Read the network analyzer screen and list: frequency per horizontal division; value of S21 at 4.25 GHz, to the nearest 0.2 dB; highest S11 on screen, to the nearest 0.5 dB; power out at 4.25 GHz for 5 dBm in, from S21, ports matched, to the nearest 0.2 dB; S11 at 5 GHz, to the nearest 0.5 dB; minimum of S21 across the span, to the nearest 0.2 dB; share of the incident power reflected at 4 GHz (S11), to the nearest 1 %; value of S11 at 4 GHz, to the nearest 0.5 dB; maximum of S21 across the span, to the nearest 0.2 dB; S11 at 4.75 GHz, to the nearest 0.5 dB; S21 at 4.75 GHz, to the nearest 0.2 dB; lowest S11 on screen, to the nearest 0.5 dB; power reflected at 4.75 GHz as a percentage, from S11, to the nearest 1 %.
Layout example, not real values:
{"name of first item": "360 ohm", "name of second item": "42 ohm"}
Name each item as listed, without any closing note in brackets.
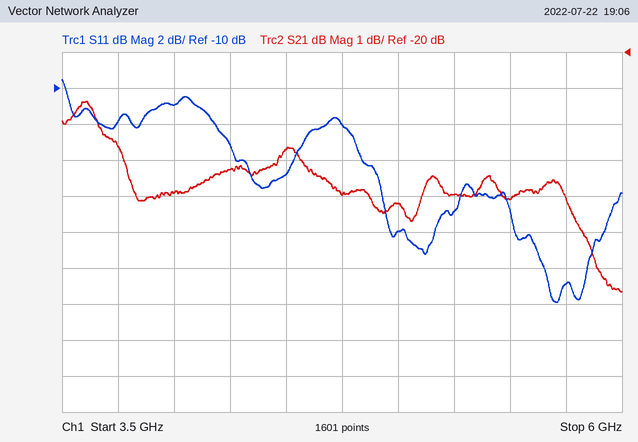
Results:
{"frequency per horizontal division": "250 MHz", "value of S21 at 4.25 GHz, to the nearest 0.2 dB": "-23.2 dB", "highest S11 on screen, to the nearest 0.5 dB": "-9.5 dB", "power out at 4.25 GHz for 5 dBm in, from S21, ports matched, to the nearest 0.2 dB": "-18.2 dBm", "S11 at 5 GHz, to the nearest 0.5 dB": "-18.0 dB", "minimum of S21 across the span, to the nearest 0.2 dB": "-26.6 dB", "share of the incident power reflected at 4 GHz (S11), to the nearest 1 %": "8 %", "value of S11 at 4 GHz, to the nearest 0.5 dB": "-11.0 dB", "maximum of S21 across the span, to the nearest 0.2 dB": "-21.4 dB", "S11 at 4.75 GHz, to the nearest 0.5 dB": "-12.0 dB", "S21 at 4.75 GHz, to the nearest 0.2 dB": "-24.0 dB", "lowest S11 on screen, to the nearest 0.5 dB": "-22.0 dB", "power reflected at 4.75 GHz as a percentage, from S11, to the nearest 1 %": "6 %"}
